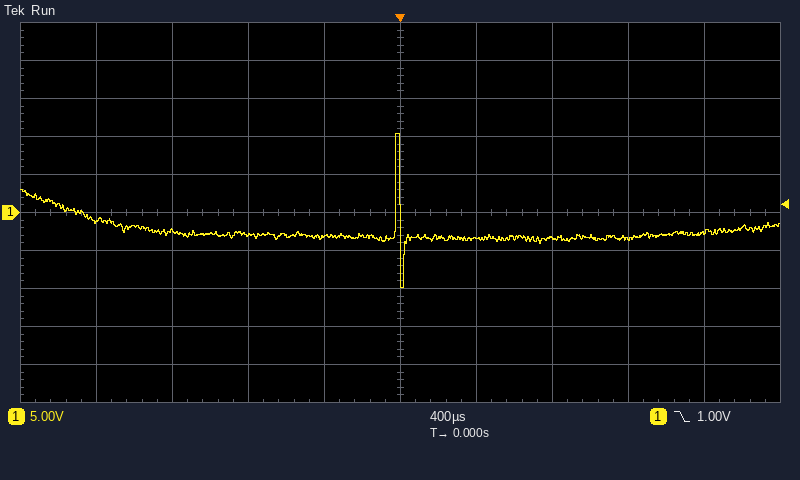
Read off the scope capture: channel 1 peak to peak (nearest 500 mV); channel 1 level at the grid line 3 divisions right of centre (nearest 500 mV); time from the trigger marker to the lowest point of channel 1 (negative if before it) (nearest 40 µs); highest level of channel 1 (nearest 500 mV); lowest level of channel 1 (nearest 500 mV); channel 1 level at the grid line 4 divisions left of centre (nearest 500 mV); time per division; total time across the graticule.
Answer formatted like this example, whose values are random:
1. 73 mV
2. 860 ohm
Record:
1. 20.5 V
2. -3.5 V
3. 0 µs
4. 10.5 V
5. -10.0 V
6. -1.0 V
7. 400 µs
8. 4 ms
